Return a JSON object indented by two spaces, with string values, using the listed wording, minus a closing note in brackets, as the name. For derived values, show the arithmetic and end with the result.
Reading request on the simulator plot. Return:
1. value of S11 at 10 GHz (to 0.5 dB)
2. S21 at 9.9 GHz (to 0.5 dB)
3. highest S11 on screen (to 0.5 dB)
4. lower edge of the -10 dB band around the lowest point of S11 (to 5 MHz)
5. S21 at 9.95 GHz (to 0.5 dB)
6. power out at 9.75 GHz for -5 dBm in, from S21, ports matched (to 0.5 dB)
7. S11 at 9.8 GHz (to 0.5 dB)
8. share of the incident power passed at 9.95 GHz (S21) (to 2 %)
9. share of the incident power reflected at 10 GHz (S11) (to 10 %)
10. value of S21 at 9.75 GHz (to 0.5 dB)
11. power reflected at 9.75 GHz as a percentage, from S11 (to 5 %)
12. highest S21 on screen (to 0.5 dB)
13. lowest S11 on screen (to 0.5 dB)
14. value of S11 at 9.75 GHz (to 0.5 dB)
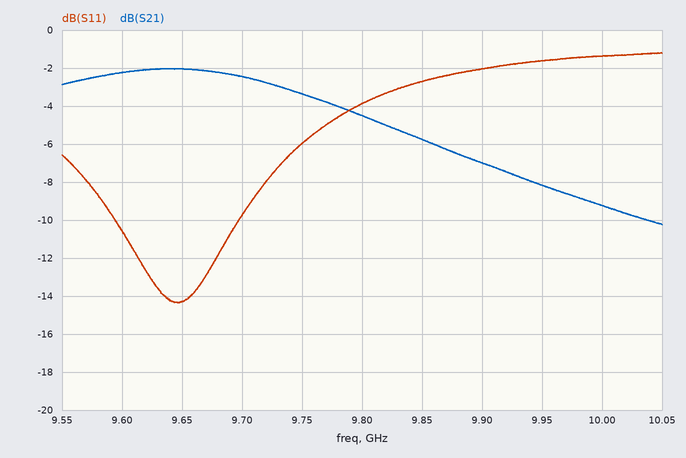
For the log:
{
  "value of S11 at 10 GHz": "-1.5 dB",
  "S21 at 9.9 GHz": "-7.0 dB",
  "highest S11 on screen": "-1.0 dB",
  "lower edge of the -10 dB band around the lowest point of S11": "9.595 GHz",
  "S21 at 9.95 GHz": "-8.0 dB",
  "power out at 9.75 GHz for -5 dBm in, from S21, ports matched": "-5 dBm + (-3.5 dB) = -8.5 dBm",
  "S11 at 9.8 GHz": "-4.0 dB",
  "share of the incident power passed at 9.95 GHz (S21)": "10^(-8/10) ≈ 16 %",
  "share of the incident power reflected at 10 GHz (S11)": "10^(-1.5/10) ≈ 70.8 %, so 70 % to the nearest 10 %",
  "value of S21 at 9.75 GHz": "-3.5 dB",
  "power reflected at 9.75 GHz as a percentage, from S11": "10^(-6/10) ≈ 25 %",
  "highest S21 on screen": "-2.0 dB",
  "lowest S11 on screen": "-14.5 dB",
  "value of S11 at 9.75 GHz": "-6.0 dB"
}
